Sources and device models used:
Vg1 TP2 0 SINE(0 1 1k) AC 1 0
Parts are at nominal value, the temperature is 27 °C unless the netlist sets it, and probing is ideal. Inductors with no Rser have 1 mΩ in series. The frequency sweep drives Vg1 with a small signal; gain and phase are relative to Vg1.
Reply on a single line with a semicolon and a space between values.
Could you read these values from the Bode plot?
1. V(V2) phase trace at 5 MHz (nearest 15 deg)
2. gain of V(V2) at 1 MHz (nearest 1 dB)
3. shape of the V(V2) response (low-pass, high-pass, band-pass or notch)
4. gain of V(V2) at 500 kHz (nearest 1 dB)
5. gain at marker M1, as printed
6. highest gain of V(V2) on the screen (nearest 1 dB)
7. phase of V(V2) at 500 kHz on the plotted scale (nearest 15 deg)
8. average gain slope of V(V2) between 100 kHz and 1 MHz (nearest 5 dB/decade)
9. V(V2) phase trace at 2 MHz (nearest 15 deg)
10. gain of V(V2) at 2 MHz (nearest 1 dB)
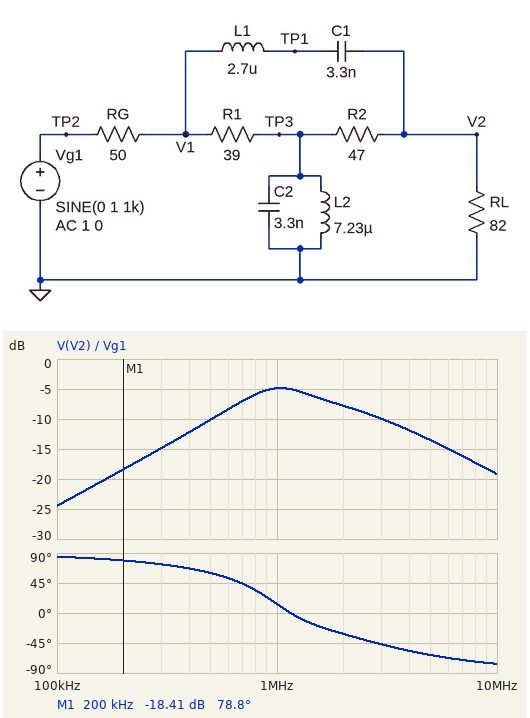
-60 deg; -5 dB; band-pass; -10 dB; -18.41 dB; -5 dB; 60 deg; 20 dB/decade; -30 deg; -8 dB
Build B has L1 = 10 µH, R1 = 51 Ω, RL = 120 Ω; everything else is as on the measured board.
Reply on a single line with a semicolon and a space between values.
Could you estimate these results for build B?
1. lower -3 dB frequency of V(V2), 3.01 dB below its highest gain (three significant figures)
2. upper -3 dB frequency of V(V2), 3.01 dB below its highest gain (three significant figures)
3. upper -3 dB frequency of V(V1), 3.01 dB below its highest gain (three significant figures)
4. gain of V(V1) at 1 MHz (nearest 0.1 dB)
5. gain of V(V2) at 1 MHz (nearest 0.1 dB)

616 kHz; 1.56 MHz; 2.00 MHz; -2.9 dB; -3.2 dB
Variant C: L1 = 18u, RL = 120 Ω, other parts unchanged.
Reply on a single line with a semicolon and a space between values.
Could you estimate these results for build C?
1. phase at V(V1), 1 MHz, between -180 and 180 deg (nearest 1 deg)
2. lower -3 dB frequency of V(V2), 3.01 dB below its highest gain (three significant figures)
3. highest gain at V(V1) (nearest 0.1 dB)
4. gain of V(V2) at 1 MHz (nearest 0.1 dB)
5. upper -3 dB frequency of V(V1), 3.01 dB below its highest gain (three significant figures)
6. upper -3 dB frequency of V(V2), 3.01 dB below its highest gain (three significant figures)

6 deg; 491 kHz; -2.3 dB; -4.8 dB; 1.84 MHz; 1.57 MHz
